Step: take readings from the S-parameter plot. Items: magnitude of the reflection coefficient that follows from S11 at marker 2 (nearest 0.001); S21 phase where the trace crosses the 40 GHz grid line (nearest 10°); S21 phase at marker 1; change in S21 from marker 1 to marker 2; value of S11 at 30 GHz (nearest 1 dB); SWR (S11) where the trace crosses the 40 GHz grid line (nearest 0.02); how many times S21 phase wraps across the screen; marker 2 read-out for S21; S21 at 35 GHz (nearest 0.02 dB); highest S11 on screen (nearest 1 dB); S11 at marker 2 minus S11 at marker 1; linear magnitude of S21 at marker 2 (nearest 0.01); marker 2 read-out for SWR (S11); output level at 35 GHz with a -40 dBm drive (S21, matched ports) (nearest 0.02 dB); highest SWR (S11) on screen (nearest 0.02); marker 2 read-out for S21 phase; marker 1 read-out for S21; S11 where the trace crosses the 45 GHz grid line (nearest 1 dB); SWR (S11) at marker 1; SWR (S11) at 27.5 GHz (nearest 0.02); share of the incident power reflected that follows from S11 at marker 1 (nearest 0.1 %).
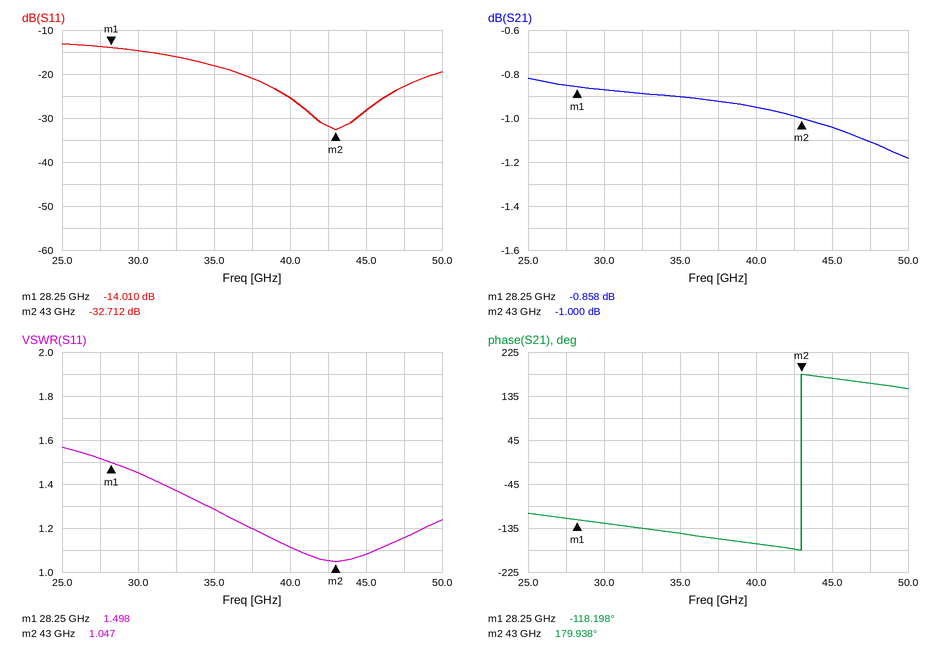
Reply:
0.023
-170°
-118.198°
-0.142 dB
-15 dB
1.12
1
-1.000 dB
-0.90 dB
-13 dB
-18.702 dB
0.89
1.047
-40.90 dBm
1.56
179.938°
-0.858 dB
-28 dB
1.498
1.52
4.0 %
